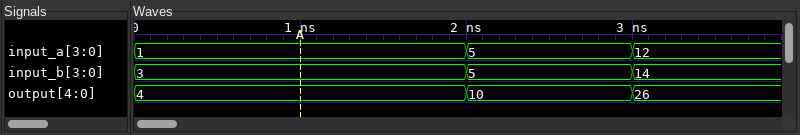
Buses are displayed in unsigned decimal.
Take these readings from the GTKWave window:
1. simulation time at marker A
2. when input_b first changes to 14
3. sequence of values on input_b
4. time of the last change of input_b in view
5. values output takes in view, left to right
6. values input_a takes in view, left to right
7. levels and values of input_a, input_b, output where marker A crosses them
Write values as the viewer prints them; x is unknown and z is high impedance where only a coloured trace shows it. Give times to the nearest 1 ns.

1 ns
3 ns
3, 5, 14
3 ns
4, 10, 26
1, 5, 12
input_a=1, input_b=3, output=4
